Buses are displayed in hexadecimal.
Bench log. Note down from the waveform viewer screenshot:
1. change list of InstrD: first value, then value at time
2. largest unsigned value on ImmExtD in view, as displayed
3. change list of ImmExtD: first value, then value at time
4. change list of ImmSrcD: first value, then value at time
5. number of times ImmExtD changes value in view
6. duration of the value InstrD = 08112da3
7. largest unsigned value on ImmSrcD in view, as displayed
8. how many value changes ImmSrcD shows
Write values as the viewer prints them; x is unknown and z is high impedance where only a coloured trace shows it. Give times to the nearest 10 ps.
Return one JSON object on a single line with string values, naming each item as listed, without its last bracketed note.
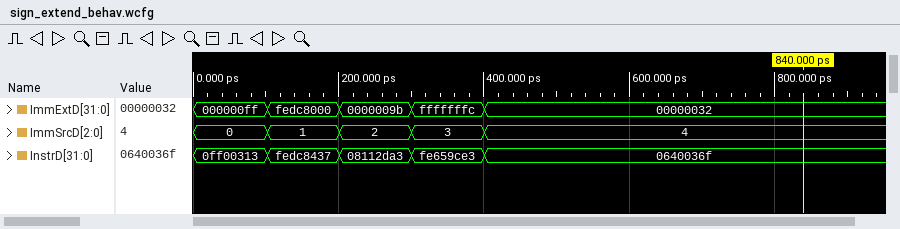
{"change list of InstrD: first value, then value at time": "0ff00313, fedc8437 at 100 ps, 08112da3 at 200 ps, fe659ce3 at 300 ps, 0640036f at 400 ps", "largest unsigned value on ImmExtD in view, as displayed": "fffffffc", "change list of ImmExtD: first value, then value at time": "000000ff, fedc8000 at 100 ps, 0000009b at 200 ps, fffffffc at 300 ps, 00000032 at 400 ps", "change list of ImmSrcD: first value, then value at time": "0, 1 at 100 ps, 2 at 200 ps, 3 at 300 ps, 4 at 400 ps", "number of times ImmExtD changes value in view": "4", "duration of the value InstrD = 08112da3": "100 ps", "largest unsigned value on ImmSrcD in view, as displayed": "4", "how many value changes ImmSrcD shows": "4"}
